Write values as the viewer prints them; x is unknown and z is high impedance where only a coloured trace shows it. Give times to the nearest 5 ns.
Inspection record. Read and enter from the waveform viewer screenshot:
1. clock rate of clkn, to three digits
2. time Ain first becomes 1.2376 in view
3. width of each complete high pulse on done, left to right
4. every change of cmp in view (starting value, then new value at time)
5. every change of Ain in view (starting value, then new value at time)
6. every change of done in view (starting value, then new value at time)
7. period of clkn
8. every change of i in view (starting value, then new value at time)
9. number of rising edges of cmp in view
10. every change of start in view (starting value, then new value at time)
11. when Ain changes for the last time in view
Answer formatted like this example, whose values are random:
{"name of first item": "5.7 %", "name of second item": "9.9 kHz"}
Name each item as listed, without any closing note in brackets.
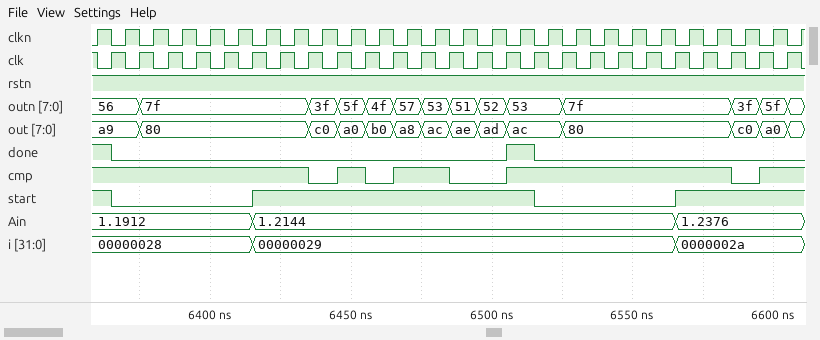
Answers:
{"clock rate of clkn, to three digits": "100 MHz", "time Ain first becomes 1.2376 in view": "6565 ns", "width of each complete high pulse on done, left to right": "10 ns", "every change of cmp in view": "1, 0 at 6435 ns, 1 at 6445 ns, 0 at 6455 ns, 1 at 6465 ns, 0 at 6485 ns, 1 at 6505 ns, 0 at 6585 ns, 1 at 6595 ns", "every change of Ain in view": "1.1912, 1.2144 at 6415 ns, 1.2376 at 6565 ns", "every change of done in view": "1, 0 at 6365 ns, 1 at 6505 ns, 0 at 6515 ns", "period of clkn": "10 ns", "every change of i in view": "00000028, 00000029 at 6415 ns, 0000002a at 6565 ns", "number of rising edges of cmp in view": "4", "every change of start in view": "1, 0 at 6365 ns, 1 at 6415 ns, 0 at 6515 ns, 1 at 6565 ns", "when Ain changes for the last time in view": "6565 ns"}
